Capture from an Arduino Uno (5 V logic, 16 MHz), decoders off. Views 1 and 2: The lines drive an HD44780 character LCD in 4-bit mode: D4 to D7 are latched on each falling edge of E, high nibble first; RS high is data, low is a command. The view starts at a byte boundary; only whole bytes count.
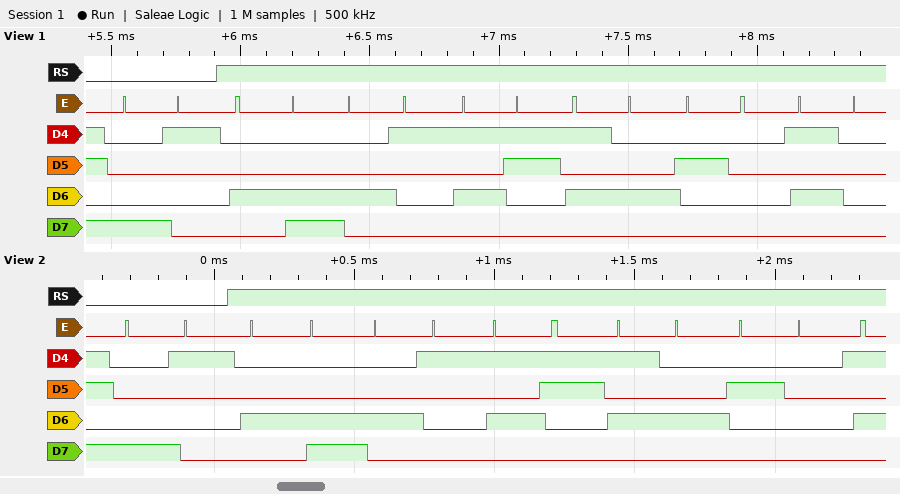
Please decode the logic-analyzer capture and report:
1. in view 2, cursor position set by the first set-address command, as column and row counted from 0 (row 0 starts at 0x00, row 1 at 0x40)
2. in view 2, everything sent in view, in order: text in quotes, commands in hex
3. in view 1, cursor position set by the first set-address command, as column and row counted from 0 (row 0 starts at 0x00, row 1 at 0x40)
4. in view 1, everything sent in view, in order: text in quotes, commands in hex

column 1, row 0
0x81 "LAST "
column 1, row 0
0x81 "LAST P"
